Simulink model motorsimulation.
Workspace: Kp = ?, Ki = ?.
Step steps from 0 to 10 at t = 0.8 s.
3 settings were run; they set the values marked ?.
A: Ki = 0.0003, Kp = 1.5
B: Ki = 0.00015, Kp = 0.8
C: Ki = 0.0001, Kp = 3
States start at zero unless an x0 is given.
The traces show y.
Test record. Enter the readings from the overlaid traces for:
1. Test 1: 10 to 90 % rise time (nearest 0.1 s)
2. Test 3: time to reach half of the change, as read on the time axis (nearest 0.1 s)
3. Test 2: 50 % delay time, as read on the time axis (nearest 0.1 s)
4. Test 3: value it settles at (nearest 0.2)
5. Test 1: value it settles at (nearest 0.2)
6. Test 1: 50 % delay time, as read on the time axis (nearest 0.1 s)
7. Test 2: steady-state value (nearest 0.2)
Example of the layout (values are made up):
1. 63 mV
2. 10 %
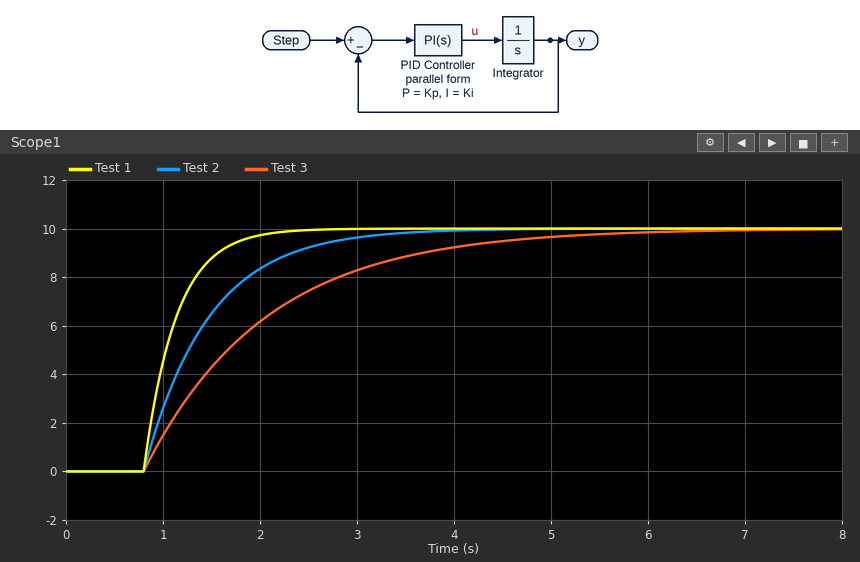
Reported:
1. 0.7 s
2. 1.7 s
3. 1.3 s
4. 10.0
5. 10.0
6. 1.0 s
7. 10.0
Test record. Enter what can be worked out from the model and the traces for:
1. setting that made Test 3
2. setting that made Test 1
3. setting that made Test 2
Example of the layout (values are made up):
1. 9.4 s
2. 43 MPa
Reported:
1. B
2. C
3. A
